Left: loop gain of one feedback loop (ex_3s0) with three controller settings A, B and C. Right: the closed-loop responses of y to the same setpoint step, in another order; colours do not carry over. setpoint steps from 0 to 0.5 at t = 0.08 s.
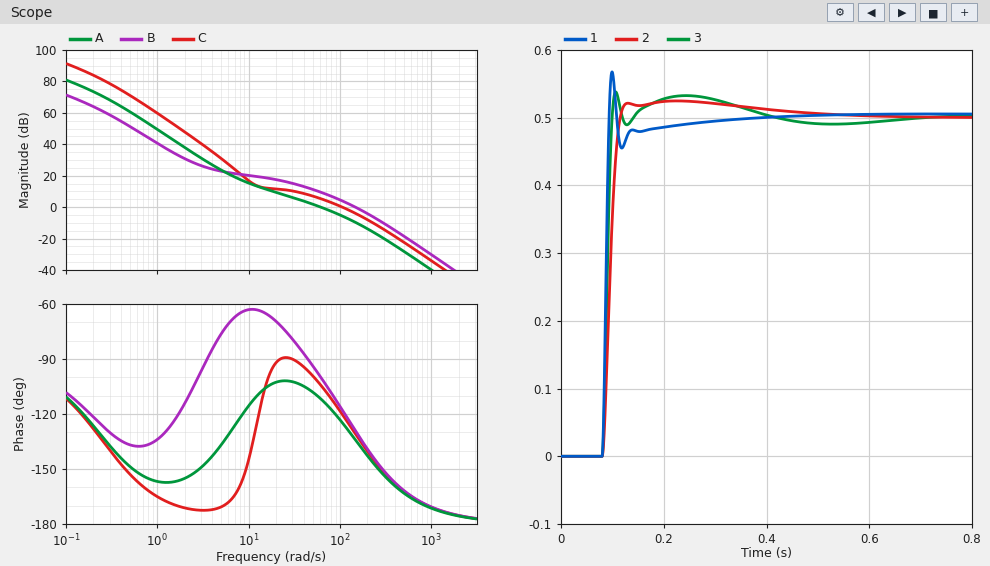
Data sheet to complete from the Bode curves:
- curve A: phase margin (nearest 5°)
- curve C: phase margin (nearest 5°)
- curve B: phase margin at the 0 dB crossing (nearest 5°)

70°
60°
50°
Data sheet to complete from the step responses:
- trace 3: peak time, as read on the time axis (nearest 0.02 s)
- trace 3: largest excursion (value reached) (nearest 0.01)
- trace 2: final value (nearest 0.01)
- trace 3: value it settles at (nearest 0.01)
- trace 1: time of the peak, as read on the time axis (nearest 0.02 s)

0.10 s
0.54
0.50
0.50
0.10 s
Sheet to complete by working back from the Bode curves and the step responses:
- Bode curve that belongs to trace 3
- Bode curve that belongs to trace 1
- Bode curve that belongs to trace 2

C
B
A
